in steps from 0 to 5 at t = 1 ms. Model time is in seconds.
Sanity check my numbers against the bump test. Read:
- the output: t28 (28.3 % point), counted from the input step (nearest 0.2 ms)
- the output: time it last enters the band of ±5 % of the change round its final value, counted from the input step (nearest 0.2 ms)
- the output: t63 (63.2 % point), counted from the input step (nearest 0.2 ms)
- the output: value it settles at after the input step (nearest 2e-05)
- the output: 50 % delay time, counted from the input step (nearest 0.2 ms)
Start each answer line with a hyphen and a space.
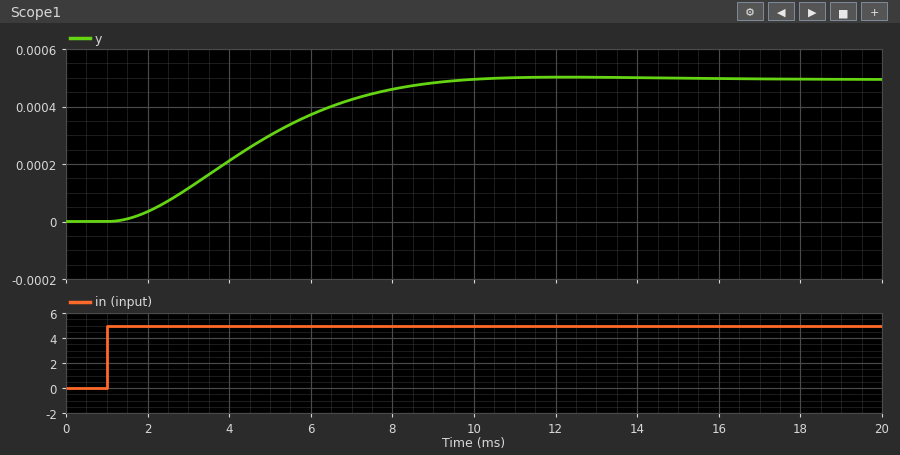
- 2.2 ms
- 7.4 ms
- 4.2 ms
- 0.00050
- 3.4 ms
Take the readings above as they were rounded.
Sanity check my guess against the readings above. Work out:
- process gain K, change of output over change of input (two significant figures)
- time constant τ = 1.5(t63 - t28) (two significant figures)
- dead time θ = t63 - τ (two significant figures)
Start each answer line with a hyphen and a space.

- 0.00010
- 3.0 ms
- 1.2 ms
